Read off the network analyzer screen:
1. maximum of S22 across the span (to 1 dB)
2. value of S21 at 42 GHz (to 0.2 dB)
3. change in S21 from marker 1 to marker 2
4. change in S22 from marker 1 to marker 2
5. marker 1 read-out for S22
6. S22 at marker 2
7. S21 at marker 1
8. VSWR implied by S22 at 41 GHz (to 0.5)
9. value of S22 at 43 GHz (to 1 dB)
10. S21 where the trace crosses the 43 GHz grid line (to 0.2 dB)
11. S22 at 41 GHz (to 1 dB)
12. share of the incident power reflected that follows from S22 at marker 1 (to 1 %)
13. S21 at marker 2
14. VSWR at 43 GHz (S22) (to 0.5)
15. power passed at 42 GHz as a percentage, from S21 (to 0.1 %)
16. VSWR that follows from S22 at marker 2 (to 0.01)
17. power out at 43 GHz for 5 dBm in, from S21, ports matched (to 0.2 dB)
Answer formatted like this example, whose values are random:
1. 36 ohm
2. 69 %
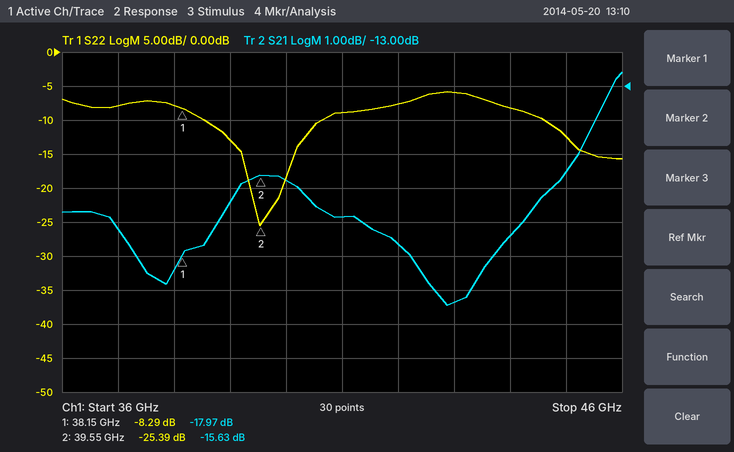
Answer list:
1. -6 dB
2. -17.6 dB
3. 2.34 dB
4. -17.10 dB
5. -8.29 dB
6. -25.39 dB
7. -17.97 dB
8. 2.0
9. -6 dB
10. -19.4 dB
11. -9 dB
12. 15 %
13. -15.63 dB
14. 3.0
15. 1.7 %
16. 1.11
17. -14.4 dBm
